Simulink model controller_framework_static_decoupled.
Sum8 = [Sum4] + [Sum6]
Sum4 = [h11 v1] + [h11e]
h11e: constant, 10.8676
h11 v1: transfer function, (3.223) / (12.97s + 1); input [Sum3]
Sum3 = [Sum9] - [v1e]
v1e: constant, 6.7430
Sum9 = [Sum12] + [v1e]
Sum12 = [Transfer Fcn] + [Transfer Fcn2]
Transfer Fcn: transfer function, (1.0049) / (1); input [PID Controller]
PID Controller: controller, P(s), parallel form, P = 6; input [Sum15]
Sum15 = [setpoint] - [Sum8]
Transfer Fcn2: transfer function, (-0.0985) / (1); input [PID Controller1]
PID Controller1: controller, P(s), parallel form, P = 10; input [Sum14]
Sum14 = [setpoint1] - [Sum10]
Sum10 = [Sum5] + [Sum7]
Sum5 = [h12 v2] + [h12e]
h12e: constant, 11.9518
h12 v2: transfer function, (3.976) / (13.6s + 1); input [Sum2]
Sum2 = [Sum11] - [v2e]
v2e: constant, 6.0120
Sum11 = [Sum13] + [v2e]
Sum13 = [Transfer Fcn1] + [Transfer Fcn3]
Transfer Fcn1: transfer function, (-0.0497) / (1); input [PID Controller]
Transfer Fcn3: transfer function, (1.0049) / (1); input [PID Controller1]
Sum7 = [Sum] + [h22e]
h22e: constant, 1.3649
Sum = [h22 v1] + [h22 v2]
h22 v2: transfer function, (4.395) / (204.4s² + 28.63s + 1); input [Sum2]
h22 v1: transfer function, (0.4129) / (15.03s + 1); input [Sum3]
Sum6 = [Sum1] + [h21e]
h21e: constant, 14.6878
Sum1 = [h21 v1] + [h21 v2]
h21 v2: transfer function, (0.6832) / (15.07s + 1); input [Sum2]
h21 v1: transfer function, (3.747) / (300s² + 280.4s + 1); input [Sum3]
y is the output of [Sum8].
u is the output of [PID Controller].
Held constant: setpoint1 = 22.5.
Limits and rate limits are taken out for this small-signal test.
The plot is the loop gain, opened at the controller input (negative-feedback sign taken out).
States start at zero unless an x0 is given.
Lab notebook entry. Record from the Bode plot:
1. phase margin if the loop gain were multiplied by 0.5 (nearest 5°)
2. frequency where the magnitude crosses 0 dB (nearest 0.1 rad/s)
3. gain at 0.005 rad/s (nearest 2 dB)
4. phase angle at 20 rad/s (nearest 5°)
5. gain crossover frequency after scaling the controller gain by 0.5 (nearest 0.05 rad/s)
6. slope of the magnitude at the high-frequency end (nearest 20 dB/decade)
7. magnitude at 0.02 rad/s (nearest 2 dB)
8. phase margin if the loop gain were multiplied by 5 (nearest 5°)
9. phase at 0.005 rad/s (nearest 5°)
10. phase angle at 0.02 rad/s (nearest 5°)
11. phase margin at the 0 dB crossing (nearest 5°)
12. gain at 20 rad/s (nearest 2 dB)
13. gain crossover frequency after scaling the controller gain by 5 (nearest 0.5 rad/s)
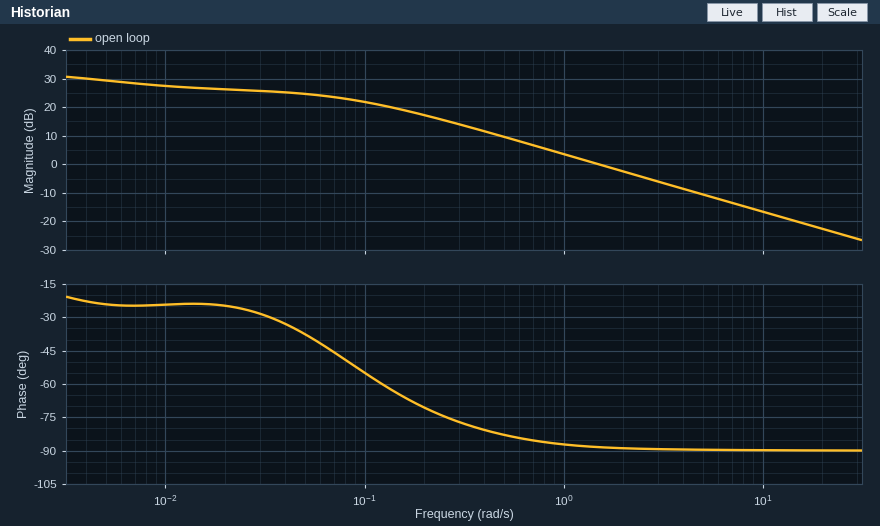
95°
1.5 rad/s
30 dB
-90°
0.75 rad/s
-20 dB/decade
26 dB
90°
-25°
-25°
90°
-22 dB
7.5 rad/s
